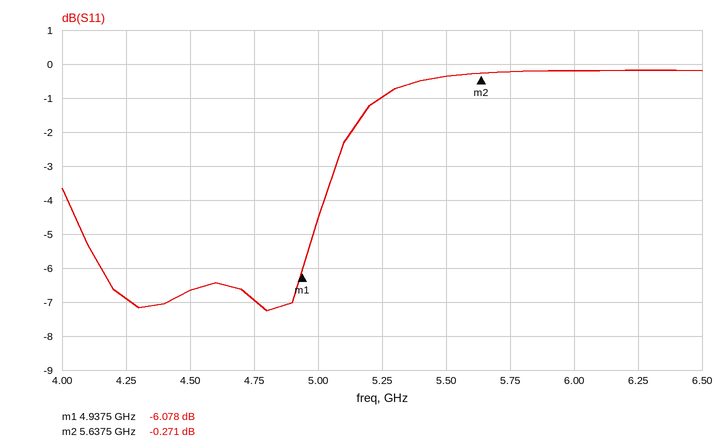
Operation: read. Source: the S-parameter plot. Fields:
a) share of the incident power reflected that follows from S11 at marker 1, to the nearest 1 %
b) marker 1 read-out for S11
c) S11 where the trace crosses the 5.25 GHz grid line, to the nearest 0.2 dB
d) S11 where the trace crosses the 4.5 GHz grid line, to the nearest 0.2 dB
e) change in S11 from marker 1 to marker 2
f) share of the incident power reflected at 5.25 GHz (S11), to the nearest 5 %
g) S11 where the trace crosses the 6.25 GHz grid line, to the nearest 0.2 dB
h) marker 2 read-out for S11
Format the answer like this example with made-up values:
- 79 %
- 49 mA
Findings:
- 25 %
- -6.078 dB
- -1.0 dB
- -6.6 dB
- 5.807 dB
- 80 %
- -0.2 dB
- -0.271 dB
